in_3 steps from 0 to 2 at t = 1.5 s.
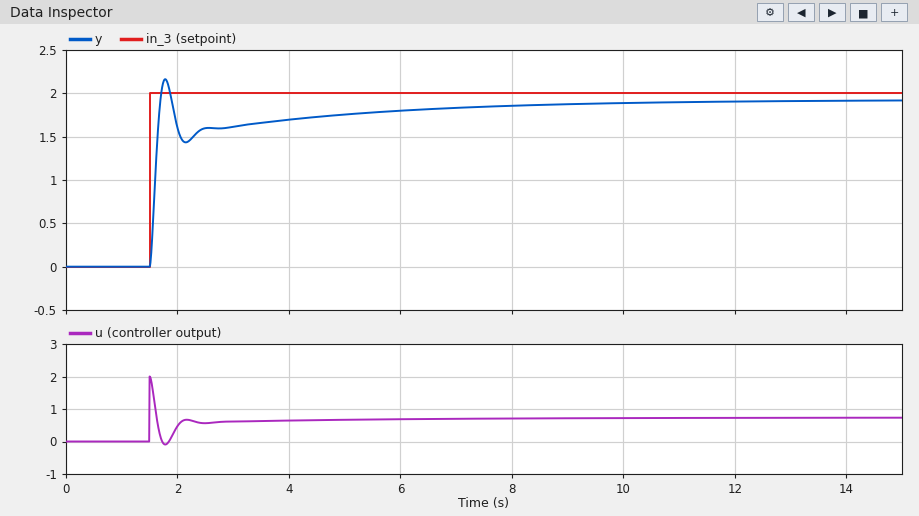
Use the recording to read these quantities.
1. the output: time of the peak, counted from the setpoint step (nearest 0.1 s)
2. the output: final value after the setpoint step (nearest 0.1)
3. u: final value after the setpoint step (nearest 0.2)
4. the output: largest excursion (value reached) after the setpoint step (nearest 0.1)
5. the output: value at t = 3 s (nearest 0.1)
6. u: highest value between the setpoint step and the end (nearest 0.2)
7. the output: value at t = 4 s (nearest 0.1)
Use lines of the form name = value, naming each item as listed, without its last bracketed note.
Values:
the output: time of the peak, counted from the setpoint step = 0.3 s
the output: final value after the setpoint step = 1.9
u: final value after the setpoint step = 0.8
the output: largest excursion (value reached) after the setpoint step = 2.2
the output: value at t = 3 s = 1.6
u: highest value between the setpoint step and the end = 2.0
the output: value at t = 4 s = 1.7
